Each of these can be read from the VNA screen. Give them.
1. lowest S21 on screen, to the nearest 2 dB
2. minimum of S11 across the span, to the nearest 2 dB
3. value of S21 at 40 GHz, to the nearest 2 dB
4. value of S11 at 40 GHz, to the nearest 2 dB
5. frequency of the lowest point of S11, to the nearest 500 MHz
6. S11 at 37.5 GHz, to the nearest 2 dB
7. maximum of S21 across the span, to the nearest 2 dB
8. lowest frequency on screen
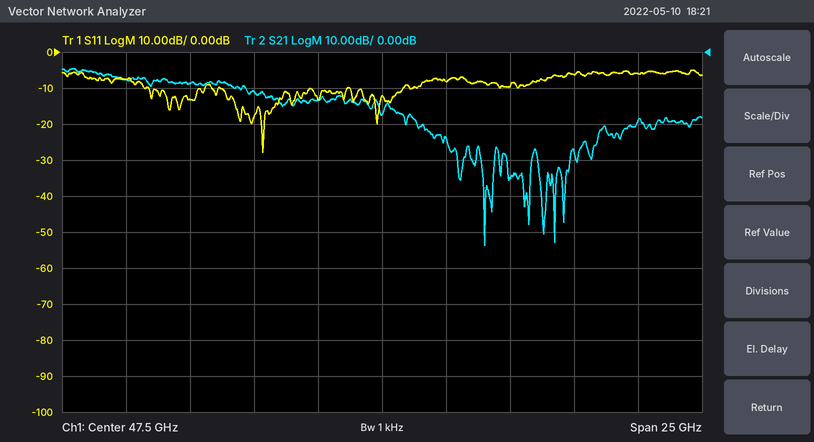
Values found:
-54 dB
-28 dB
-8 dB
-14 dB
43.0 GHz
-8 dB
-4 dB
35 GHz
